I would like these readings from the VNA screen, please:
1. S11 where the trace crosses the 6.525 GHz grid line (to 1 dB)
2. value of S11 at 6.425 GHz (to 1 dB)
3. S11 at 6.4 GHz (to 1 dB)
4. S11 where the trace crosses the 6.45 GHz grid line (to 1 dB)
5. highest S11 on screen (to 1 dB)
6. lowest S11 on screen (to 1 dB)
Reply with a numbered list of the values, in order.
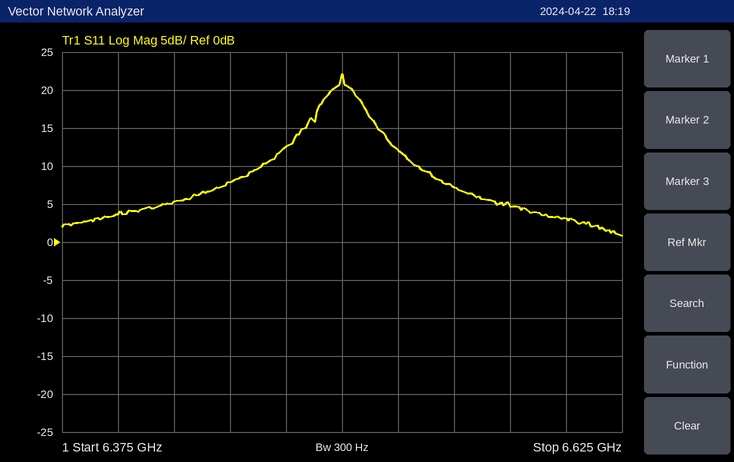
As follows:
1. 12 dB
2. 5 dB
3. 4 dB
4. 8 dB
5. 22 dB
6. 1 dB
